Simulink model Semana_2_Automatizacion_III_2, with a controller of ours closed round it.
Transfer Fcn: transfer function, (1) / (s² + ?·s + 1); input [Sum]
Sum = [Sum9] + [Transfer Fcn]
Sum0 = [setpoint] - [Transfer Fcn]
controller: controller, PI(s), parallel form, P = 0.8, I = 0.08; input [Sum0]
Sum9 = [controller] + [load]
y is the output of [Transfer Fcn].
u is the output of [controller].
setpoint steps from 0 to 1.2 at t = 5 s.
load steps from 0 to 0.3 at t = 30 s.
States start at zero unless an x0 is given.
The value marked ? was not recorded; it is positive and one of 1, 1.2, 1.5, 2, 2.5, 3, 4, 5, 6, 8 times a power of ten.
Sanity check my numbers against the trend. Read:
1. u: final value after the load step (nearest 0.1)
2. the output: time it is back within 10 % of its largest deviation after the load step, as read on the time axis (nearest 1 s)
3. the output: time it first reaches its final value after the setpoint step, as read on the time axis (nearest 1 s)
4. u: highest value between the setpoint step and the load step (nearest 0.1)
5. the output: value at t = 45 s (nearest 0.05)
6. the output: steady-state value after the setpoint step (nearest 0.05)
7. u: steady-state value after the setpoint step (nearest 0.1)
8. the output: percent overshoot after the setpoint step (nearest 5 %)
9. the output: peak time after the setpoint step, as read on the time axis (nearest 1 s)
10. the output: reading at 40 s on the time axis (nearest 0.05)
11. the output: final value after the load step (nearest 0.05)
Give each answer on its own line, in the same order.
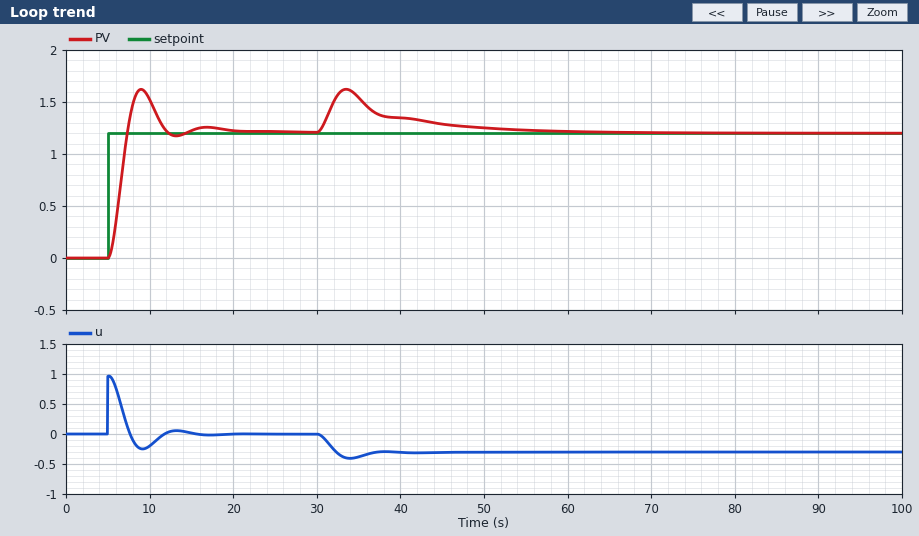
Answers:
-0.3
52 s
7 s
1.0
1.30
1.20
0.0
35 %
9 s
1.35
1.20
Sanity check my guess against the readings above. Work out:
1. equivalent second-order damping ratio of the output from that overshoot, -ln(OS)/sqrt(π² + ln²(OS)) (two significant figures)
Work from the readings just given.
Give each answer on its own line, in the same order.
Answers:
0.32
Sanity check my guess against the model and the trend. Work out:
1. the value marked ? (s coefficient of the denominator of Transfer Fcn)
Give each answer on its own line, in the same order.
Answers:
0.8
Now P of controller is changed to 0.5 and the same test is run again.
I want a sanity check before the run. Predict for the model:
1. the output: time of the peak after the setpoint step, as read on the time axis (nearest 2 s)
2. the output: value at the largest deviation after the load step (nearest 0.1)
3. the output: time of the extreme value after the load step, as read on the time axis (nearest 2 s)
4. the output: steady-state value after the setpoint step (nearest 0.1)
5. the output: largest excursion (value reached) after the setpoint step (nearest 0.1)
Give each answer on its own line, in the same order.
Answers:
10 s
1.8
34 s
1.2
1.7
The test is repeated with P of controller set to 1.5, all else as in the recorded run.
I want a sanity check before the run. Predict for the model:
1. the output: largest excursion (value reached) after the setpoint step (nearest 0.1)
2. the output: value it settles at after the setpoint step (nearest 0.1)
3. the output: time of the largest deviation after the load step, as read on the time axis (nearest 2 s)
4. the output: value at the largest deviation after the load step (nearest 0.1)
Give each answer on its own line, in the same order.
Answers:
1.7
1.2
32 s
1.5
